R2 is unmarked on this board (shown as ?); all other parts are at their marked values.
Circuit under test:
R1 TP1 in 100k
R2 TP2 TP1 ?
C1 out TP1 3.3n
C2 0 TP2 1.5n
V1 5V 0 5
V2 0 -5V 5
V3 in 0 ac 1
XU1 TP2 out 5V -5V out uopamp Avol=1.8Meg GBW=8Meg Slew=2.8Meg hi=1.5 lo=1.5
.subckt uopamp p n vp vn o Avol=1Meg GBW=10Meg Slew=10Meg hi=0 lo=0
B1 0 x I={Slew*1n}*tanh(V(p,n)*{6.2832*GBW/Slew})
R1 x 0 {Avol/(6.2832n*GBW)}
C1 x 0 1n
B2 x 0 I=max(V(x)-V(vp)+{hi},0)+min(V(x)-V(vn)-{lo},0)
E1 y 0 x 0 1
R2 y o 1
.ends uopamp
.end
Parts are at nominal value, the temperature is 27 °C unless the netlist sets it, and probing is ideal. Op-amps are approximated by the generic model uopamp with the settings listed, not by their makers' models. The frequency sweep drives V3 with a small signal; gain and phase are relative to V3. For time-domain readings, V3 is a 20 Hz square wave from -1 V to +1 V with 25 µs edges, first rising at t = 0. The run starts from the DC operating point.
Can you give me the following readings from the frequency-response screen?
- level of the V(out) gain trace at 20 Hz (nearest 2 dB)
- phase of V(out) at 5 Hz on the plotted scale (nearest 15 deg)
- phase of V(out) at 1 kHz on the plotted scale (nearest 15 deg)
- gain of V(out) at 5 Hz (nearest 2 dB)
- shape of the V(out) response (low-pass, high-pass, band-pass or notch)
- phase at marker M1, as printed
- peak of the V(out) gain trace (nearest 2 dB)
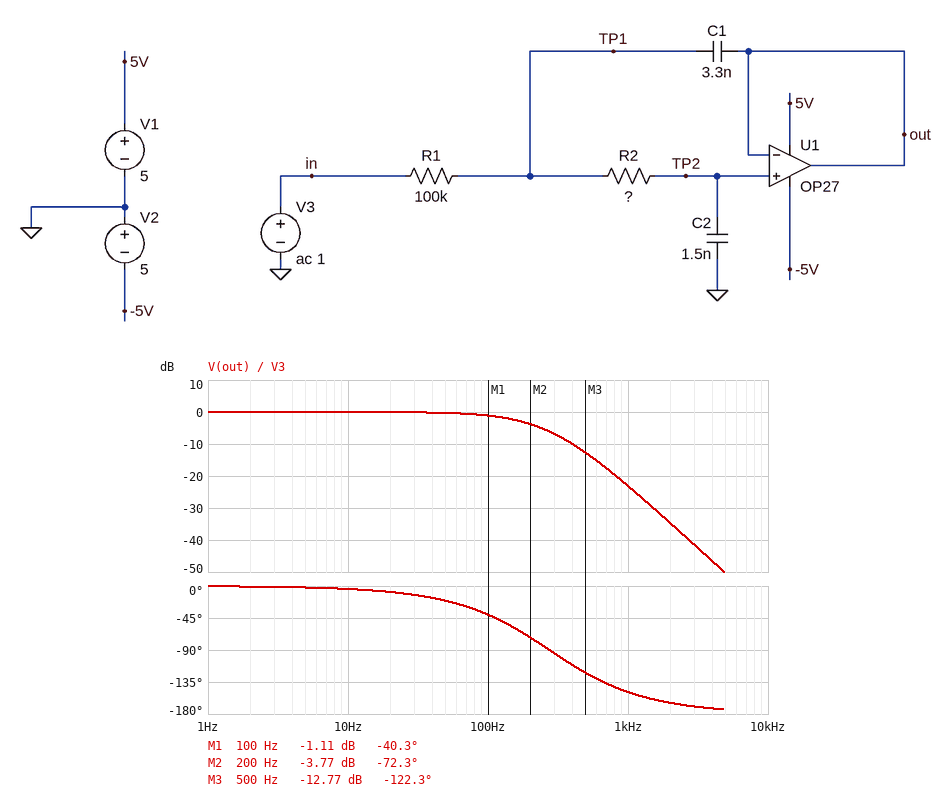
0 dB
0 deg
-150 deg
0 dB
low-pass
-40.3 deg
0 dB
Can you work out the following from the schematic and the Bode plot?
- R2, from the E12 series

680 kΩ
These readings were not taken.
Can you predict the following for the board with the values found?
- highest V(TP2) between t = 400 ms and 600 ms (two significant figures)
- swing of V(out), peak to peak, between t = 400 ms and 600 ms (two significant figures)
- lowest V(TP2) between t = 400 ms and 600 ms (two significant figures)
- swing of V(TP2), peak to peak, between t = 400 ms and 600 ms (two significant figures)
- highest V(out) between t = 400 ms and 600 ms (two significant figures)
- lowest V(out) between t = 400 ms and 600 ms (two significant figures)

1.0 V
2.0 V
-1.0 V
2.0 V
1.0 V
-1.0 V
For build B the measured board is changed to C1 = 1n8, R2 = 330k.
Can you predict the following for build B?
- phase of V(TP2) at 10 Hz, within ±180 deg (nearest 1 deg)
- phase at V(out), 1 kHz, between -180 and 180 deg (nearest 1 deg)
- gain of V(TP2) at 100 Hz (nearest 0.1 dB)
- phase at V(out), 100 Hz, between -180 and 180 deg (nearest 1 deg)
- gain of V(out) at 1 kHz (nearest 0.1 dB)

-2 deg
-122 deg
-0.4 dB
-23 deg
-13.6 dB
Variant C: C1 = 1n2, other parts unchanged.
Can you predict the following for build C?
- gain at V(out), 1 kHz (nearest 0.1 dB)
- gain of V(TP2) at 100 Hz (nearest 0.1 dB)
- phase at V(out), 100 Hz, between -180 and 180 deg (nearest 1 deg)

-18.4 dB
-1.6 dB
-38 deg
